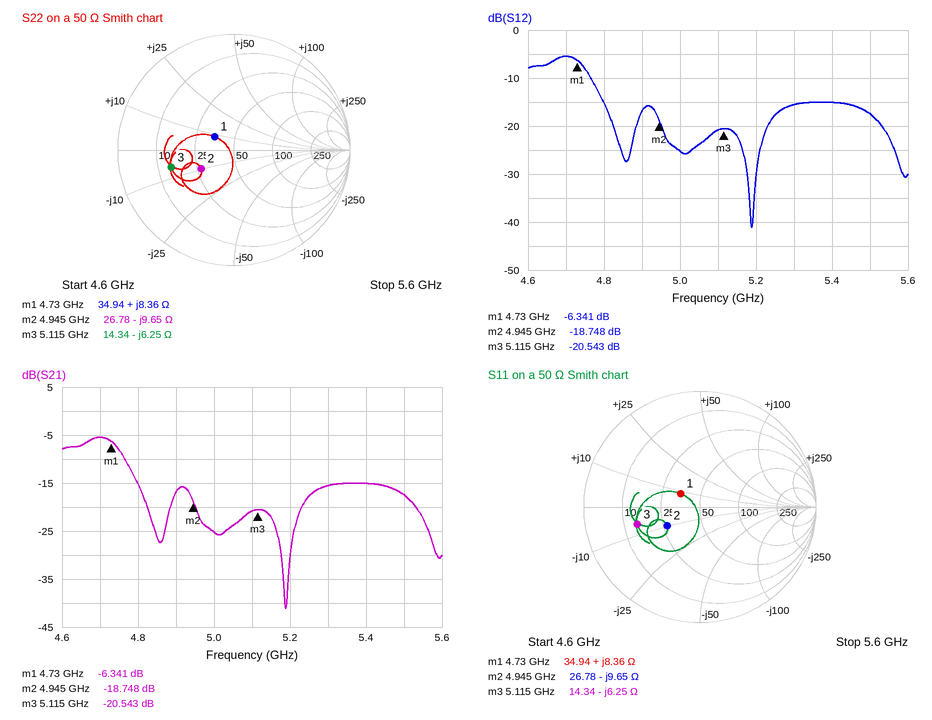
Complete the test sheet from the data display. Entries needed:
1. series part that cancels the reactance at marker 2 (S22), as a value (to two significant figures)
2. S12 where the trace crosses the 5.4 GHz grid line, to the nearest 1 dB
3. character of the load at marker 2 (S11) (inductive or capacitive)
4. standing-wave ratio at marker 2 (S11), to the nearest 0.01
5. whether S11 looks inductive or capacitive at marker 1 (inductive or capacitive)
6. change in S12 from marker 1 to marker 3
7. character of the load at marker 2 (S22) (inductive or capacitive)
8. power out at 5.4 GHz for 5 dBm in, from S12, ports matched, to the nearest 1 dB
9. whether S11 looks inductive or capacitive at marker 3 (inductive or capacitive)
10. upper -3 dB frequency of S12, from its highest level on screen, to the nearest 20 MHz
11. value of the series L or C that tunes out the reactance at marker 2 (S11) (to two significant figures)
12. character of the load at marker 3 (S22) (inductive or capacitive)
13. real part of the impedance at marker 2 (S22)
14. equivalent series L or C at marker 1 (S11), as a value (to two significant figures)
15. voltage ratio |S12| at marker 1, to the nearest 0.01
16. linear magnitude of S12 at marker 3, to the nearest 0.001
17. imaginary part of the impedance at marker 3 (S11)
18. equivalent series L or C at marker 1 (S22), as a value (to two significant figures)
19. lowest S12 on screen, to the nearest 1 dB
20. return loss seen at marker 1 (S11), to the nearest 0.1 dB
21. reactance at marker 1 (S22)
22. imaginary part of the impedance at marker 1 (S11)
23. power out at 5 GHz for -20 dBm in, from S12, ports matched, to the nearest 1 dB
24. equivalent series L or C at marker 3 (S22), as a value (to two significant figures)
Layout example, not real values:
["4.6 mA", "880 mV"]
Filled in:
["310 pH", "-15 dB", "capacitive", "1.96", "inductive", "-14.202 dB", "capacitive", "-10 dBm", "capacitive", "4.76 GHz", "310 pH", "capacitive", "26.78 Ω", "280 pH", "0.48", "0.094", "-6.25 Ω", "280 pH", "-41 dB", "13.9 dB", "+8.36 Ω", "+8.36 Ω", "-45 dBm", "5.0 pF"]
